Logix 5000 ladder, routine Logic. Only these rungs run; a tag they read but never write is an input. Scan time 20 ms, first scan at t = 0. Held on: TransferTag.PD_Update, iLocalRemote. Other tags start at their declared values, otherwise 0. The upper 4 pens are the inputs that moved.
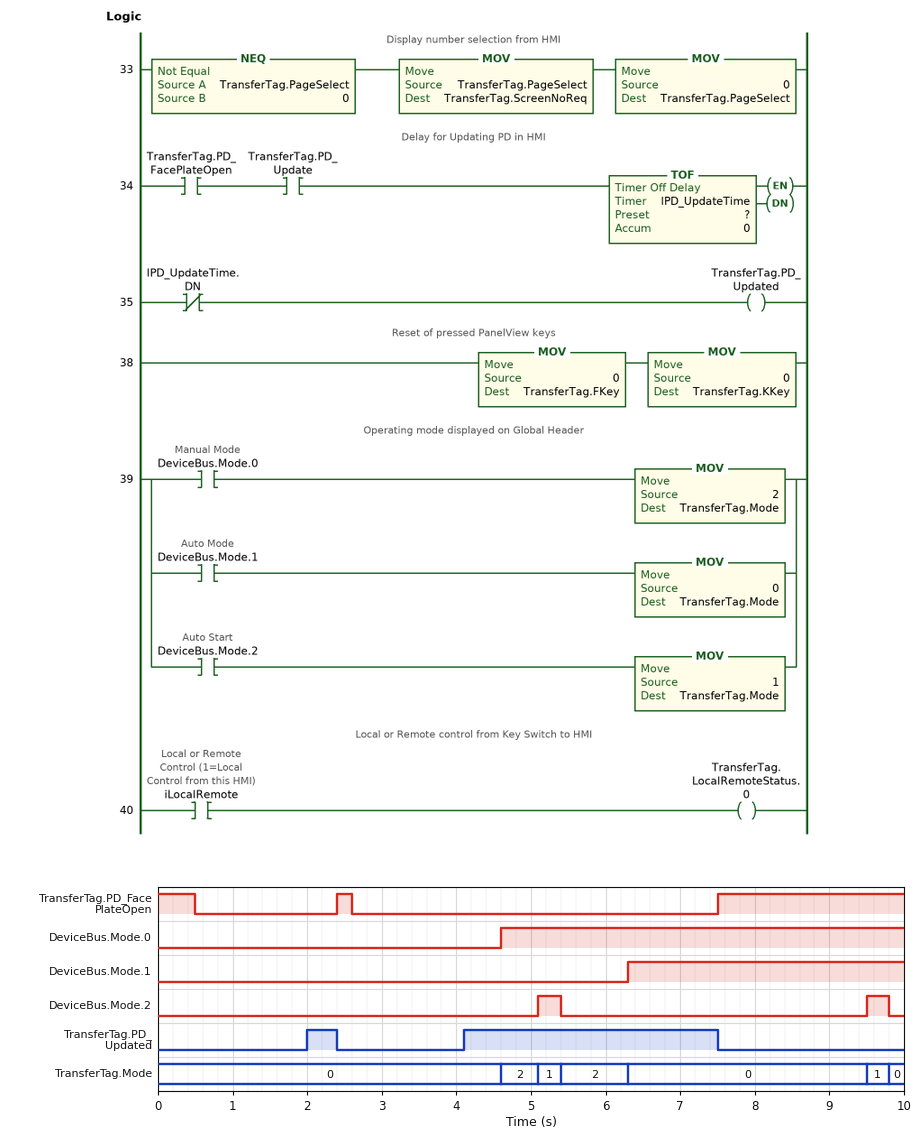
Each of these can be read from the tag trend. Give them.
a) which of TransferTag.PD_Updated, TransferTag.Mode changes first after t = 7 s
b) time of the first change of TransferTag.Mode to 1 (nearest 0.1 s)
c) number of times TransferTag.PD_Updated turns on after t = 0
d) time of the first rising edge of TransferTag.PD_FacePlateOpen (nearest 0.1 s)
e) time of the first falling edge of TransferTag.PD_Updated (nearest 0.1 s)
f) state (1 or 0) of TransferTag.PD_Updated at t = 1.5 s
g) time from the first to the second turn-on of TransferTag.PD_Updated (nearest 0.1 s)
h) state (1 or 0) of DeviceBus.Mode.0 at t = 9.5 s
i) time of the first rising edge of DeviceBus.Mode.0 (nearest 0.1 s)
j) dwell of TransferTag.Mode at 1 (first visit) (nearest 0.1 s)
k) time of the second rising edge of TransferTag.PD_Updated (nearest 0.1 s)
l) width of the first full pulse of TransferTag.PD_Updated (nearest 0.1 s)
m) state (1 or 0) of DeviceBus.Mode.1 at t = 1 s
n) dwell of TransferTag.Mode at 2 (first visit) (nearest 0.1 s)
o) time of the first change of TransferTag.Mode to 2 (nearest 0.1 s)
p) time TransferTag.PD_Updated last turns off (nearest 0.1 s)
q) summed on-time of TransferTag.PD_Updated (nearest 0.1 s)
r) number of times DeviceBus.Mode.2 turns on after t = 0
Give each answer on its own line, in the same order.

TransferTag.PD_Updated
5.1 s
2
2.4 s
2.4 s
0
2.1 s
1
4.6 s
0.3 s
4.1 s
0.4 s
0
0.5 s
4.6 s
7.5 s
3.8 s
2
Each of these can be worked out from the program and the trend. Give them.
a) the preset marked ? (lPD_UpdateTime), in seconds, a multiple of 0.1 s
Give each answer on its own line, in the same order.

1.5 s
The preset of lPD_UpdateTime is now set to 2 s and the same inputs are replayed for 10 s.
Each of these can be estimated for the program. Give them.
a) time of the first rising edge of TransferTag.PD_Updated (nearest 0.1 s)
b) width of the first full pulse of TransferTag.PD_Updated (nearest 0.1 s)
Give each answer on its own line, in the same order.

4.6 s
2.9 s
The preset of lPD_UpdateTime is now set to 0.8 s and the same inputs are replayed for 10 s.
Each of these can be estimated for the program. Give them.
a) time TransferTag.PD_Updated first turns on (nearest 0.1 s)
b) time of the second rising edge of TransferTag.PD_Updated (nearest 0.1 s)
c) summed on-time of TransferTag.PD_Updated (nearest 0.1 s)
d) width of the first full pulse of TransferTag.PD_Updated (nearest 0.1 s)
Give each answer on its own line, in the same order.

1.3 s
3.4 s
5.2 s
1.1 s
